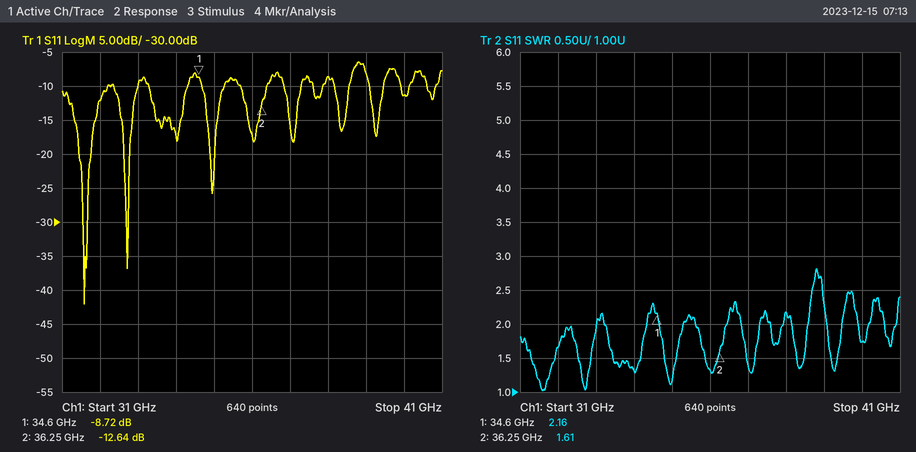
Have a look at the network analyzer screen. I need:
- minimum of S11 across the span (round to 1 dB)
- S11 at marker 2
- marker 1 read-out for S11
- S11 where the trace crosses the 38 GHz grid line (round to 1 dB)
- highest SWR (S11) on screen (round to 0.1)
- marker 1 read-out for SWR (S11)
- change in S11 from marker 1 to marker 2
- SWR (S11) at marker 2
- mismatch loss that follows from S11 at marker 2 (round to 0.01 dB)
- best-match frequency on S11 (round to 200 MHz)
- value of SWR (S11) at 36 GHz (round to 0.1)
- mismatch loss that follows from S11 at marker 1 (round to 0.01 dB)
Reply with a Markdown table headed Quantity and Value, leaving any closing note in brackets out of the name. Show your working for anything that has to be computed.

| Quantity | Value |
|---|---|
| minimum of S11 across the span | -42 dB |
| S11 at marker 2 | -12.64 dB |
| marker 1 read-out for S11 | -8.72 dB |
| S11 where the trace crosses the 38 GHz grid line | -9 dB |
| highest SWR (S11) on screen | 2.8 |
| marker 1 read-out for SWR | 2.16 |
| change in S11 from marker 1 to marker 2 | -12.64 − (-8.72) = -3.92 dB |
| SWR (S11) at marker 2 | 1.61 |
| mismatch loss that follows from S11 at marker 2 | −10 log10(1 − 10^(-12.64/10)) ≈ 0.24 dB |
| best-match frequency on S11 | 31.6 GHz |
| value of SWR (S11) at 36 GHz | 1.3 |
| mismatch loss that follows from S11 at marker 1 | −10 log10(1 − 10^(-8.72/10)) ≈ 0.63 dB |
